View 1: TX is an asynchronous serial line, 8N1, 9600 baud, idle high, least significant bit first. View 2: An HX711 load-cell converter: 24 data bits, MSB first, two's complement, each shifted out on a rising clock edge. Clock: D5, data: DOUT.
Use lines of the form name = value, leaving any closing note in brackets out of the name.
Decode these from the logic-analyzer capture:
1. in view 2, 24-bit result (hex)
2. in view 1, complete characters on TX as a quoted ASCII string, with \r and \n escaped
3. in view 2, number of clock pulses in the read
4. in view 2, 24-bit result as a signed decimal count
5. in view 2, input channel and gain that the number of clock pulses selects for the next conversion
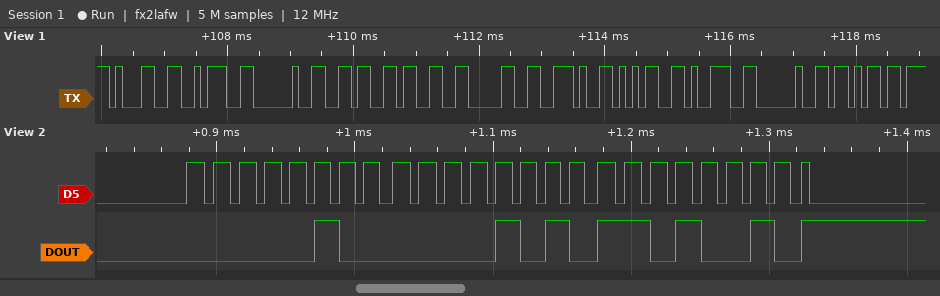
in view 2, 24-bit result = 0x040AD2
in view 1, complete characters on TX as a quoted ASCII string, with \r and \n escaped = "1: 630.59 k"
in view 2, number of clock pulses in the read = 25
in view 2, 24-bit result as a signed decimal count = 264914
in view 2, input channel and gain that the number of clock pulses selects for the next conversion = channel A, gain 128
